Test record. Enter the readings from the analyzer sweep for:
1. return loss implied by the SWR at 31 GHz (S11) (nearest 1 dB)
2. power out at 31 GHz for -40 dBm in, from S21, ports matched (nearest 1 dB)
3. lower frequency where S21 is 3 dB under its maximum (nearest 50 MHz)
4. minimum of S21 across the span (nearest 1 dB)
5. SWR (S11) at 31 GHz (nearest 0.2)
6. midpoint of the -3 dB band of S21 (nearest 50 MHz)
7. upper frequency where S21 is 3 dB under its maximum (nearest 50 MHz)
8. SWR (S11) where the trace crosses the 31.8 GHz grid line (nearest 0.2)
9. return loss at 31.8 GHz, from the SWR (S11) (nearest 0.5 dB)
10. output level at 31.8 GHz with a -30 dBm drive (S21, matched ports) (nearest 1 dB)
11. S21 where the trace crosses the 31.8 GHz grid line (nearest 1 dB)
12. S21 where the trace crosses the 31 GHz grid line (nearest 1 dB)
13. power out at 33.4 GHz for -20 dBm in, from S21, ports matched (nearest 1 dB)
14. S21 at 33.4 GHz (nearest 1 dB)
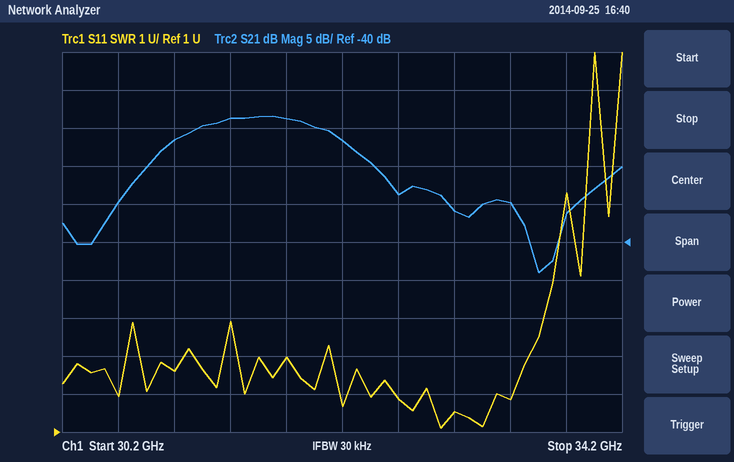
7 dB
-67 dBm
31.00 GHz
-44 dB
2.6
31.60 GHz
32.20 GHz
3.0
6.0 dB
-54 dBm
-24 dB
-27 dB
-55 dBm
-35 dB
